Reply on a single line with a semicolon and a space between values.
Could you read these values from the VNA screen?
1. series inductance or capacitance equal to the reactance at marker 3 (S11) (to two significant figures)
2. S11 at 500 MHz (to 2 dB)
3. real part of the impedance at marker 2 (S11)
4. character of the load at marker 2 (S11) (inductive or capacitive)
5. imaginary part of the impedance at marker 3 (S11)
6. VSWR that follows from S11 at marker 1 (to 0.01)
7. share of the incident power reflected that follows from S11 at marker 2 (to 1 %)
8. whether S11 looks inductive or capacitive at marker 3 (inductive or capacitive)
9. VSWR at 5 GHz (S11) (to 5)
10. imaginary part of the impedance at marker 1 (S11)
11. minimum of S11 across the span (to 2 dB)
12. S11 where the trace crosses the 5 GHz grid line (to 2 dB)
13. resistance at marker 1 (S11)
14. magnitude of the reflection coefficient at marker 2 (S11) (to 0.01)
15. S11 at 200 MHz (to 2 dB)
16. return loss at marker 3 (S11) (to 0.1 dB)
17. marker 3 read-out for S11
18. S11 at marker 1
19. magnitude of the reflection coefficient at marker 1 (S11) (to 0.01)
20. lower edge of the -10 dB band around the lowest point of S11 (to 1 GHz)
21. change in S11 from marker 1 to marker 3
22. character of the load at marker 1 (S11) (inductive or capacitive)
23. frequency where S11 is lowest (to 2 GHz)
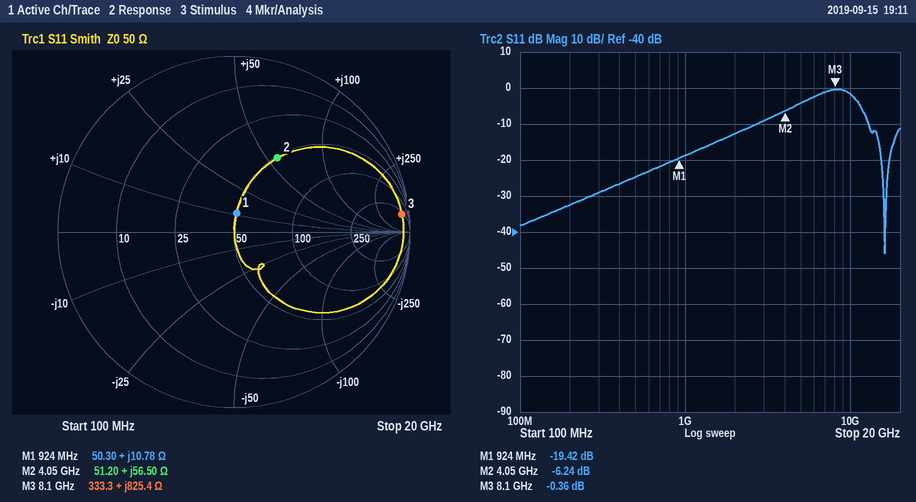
16 nH; -24 dB; 51.20 Ω; inductive; +825.4 Ω; 1.24; 24 %; inductive; 5; +10.78 Ω; -46 dB; -4 dB; 50.30 Ω; 0.49; -32 dB; 0.4 dB; -0.36 dB; -19.42 dB; 0.11; 13 GHz; 19.06 dB; inductive; 16 GHz
